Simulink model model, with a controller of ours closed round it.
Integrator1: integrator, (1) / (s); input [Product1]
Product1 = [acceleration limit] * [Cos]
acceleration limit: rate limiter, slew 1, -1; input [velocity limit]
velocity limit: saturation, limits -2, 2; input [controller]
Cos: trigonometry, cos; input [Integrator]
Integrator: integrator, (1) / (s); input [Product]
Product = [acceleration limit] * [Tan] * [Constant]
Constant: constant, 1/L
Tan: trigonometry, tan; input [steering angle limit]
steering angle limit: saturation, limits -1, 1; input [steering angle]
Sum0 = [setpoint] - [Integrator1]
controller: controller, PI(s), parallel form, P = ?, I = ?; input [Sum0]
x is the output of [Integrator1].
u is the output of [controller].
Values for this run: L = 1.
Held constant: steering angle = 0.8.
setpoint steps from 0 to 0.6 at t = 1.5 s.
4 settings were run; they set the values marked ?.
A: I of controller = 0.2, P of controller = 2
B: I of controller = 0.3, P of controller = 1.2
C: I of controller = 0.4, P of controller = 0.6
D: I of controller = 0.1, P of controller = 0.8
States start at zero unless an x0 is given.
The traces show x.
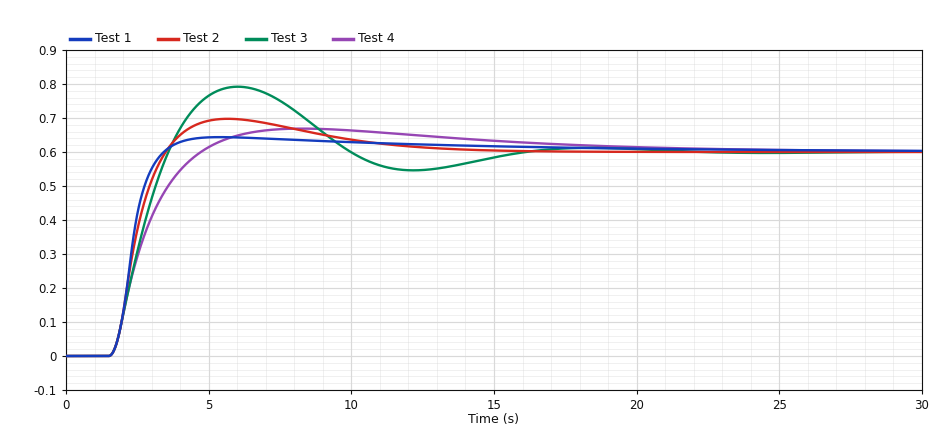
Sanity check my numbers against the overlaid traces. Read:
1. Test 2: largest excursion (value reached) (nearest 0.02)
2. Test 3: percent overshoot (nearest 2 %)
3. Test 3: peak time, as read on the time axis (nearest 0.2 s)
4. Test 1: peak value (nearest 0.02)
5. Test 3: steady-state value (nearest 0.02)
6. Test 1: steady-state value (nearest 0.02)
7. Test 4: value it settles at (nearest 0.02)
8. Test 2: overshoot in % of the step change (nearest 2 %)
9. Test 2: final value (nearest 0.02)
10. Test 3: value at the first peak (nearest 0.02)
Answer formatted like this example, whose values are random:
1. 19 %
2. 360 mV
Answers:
1. 0.70
2. 32 %
3. 6.0 s
4. 0.64
5. 0.60
6. 0.60
7. 0.60
8. 16 %
9. 0.60
10. 0.80
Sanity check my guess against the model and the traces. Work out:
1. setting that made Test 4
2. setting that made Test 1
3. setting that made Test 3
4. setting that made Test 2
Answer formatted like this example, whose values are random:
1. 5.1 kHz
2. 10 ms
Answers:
1. D
2. A
3. C
4. B
